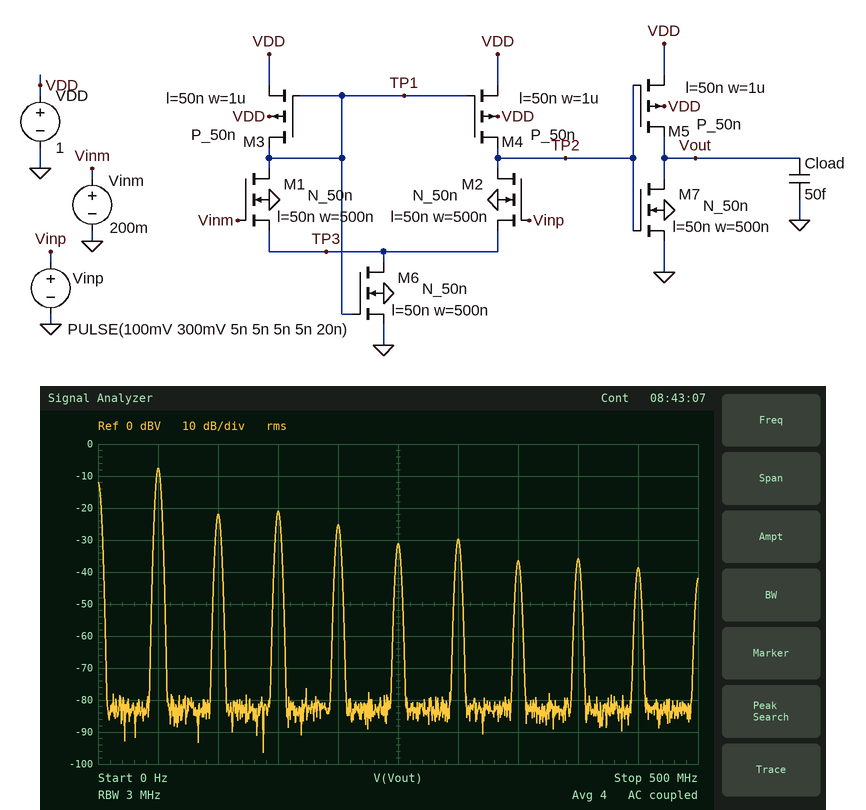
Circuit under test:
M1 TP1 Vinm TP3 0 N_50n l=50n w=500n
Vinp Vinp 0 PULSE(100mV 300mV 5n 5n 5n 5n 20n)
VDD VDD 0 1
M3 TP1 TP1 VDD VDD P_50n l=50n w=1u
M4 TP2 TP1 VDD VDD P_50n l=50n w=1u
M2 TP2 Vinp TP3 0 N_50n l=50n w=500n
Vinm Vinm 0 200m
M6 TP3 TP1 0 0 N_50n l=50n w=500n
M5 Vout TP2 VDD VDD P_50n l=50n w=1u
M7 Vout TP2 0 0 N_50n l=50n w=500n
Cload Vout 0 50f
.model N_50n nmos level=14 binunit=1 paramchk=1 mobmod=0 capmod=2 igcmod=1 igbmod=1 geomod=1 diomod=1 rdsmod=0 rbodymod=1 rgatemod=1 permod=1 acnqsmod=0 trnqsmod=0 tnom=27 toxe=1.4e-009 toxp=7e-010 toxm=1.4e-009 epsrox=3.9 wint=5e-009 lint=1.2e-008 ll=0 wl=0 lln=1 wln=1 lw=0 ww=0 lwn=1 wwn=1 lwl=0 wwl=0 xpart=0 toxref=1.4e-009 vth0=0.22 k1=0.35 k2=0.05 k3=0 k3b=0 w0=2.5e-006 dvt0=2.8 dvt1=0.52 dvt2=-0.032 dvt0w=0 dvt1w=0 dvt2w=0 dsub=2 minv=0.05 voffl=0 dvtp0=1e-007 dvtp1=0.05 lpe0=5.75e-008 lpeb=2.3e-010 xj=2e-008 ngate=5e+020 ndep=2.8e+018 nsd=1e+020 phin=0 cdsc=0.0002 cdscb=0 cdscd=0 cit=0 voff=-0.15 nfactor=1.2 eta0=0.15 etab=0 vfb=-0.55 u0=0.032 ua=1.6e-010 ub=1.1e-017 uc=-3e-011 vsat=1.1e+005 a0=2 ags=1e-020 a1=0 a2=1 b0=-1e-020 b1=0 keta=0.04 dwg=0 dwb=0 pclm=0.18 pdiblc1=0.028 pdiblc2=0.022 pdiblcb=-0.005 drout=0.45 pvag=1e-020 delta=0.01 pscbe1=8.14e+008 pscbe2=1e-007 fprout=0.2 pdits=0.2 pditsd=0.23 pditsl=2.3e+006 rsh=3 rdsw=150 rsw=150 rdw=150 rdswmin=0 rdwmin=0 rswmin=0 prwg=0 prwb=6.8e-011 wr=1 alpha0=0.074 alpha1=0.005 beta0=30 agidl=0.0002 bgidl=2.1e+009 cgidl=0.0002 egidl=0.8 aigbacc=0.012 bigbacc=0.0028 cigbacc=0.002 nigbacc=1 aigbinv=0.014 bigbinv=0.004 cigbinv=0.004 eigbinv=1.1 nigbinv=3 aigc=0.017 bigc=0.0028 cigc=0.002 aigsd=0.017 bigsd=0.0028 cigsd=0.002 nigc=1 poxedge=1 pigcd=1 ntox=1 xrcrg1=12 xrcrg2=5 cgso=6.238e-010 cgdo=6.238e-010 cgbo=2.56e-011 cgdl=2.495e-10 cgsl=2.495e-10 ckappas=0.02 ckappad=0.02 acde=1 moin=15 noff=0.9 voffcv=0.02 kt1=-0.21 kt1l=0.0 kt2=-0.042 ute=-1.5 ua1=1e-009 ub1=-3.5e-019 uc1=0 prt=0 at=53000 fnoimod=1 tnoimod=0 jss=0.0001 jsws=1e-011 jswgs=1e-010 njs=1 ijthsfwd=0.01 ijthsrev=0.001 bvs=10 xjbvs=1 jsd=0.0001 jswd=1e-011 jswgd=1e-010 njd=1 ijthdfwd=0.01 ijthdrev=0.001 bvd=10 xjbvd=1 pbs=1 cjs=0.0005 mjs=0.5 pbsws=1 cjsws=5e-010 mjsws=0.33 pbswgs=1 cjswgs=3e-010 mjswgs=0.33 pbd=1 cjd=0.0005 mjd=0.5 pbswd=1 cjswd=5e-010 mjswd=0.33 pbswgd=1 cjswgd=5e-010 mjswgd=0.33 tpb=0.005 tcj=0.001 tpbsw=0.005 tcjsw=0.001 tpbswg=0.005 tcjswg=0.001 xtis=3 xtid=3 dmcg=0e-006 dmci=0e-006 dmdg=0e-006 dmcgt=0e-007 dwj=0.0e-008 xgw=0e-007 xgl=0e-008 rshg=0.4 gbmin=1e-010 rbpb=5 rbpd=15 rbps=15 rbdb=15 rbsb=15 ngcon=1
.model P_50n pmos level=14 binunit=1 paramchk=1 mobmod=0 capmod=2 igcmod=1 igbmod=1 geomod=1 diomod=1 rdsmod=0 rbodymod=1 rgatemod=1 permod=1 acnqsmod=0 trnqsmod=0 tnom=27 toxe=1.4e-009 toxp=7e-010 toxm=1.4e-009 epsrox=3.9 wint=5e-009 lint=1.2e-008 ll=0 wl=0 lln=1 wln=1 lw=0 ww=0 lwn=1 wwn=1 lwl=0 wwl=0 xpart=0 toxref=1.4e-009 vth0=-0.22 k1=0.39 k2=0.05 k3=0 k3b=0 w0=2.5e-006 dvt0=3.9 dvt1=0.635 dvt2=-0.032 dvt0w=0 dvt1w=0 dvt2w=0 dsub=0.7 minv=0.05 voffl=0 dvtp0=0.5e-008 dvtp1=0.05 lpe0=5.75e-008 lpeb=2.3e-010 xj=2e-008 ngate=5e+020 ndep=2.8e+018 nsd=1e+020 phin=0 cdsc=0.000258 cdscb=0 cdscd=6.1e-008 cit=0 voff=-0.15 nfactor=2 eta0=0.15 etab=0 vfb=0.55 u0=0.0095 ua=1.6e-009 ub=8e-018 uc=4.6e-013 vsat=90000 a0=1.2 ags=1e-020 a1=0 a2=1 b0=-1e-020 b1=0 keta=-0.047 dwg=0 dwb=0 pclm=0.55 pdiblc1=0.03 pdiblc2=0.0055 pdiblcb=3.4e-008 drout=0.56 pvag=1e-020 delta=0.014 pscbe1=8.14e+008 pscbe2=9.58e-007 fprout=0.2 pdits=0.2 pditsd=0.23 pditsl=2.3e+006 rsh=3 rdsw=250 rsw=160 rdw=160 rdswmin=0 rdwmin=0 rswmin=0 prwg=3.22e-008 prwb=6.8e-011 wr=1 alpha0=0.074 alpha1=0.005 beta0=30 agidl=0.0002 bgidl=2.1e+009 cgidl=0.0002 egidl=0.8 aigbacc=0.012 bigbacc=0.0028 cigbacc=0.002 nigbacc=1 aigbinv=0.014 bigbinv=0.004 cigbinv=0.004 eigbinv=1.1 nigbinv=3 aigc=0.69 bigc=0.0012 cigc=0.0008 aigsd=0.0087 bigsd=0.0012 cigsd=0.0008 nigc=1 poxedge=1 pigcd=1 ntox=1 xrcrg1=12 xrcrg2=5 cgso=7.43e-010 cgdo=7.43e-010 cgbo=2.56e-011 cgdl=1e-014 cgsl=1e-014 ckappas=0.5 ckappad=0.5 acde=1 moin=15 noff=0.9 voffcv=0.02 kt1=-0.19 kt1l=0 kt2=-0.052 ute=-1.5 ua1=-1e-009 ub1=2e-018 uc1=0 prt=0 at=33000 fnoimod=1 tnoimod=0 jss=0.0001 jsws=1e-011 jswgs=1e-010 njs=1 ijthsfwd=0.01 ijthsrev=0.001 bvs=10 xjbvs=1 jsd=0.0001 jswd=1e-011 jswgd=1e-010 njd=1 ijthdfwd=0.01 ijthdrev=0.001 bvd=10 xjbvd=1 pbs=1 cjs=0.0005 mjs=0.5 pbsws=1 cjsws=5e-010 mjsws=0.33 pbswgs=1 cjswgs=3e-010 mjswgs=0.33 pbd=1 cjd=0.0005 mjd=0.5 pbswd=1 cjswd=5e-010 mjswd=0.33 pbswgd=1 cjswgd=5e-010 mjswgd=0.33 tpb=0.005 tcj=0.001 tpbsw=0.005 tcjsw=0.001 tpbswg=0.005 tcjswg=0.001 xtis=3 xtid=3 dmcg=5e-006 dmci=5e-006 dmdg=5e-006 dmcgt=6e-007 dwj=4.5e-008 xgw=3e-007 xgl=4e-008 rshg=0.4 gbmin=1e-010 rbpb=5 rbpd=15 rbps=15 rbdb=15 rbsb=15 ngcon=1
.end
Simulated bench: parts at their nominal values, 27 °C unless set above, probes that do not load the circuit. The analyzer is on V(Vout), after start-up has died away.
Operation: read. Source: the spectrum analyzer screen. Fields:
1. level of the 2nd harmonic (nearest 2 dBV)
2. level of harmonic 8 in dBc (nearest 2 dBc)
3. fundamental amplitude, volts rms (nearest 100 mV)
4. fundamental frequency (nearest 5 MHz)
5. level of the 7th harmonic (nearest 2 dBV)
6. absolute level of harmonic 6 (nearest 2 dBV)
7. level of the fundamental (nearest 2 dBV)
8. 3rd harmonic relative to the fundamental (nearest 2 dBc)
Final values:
-22 dBV
-28 dBc
400 mV
50 MHz
-36 dBV
-30 dBV
-8 dBV
-14 dBc
